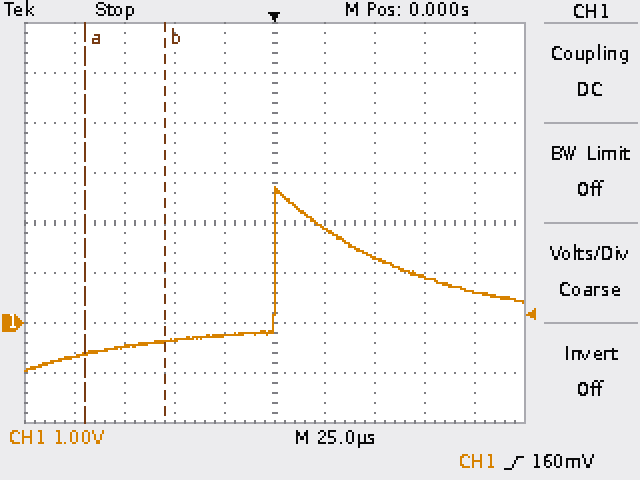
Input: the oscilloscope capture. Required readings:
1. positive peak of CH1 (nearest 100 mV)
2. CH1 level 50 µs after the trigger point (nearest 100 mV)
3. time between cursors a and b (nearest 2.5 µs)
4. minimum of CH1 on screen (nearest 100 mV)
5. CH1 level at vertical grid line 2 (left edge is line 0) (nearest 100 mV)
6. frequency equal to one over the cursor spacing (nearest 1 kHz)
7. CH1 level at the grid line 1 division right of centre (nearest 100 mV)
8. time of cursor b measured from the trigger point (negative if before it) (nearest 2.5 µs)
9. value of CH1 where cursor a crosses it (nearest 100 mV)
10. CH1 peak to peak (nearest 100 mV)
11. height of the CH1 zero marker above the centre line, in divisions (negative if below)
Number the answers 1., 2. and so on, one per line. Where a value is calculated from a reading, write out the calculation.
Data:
1. 2.7 V
2. 1.3 V
3. 40.0 µs
4. -1.0 V
5. -500 mV
6. 1 / 40.0 µs ≈ 25 kHz
7. 1.9 V
8. -55.0 µs
9. -600 mV
10. 2.7 V − (-1.0 V) = 3.7 V
11. -2.0 div
